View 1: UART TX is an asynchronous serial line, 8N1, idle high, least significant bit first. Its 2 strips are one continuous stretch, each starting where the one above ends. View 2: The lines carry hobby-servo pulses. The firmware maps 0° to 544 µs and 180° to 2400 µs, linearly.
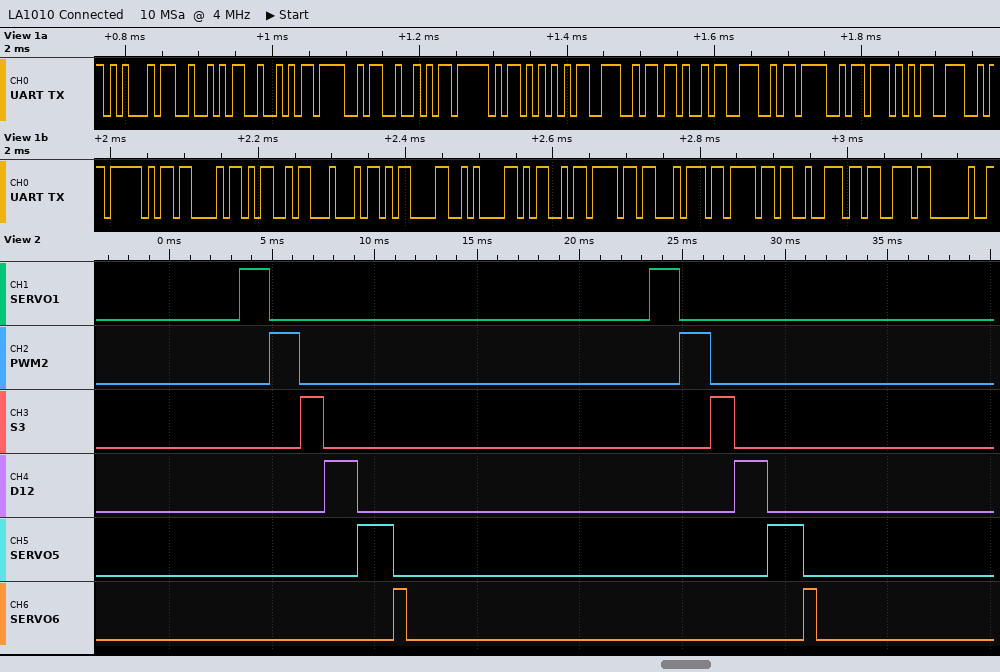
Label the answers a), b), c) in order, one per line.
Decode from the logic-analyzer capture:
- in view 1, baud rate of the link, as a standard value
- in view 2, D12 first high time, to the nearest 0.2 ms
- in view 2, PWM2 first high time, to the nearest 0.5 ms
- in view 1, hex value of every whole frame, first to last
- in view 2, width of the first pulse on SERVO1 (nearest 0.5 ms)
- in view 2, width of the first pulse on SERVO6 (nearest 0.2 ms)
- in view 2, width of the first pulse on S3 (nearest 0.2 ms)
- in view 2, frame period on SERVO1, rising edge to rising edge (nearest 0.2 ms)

a) 115200 baud
b) 1.6 ms
c) 1.5 ms
d) 45 52 52 4F 52 5F 55 4E 4B 4E 4F 57 4E 5F 43 4D 44 0D 0A 4D 6F 74 6F 72 73 20
e) 1.5 ms
f) 0.6 ms
g) 1.2 ms
h) 20.0 ms
